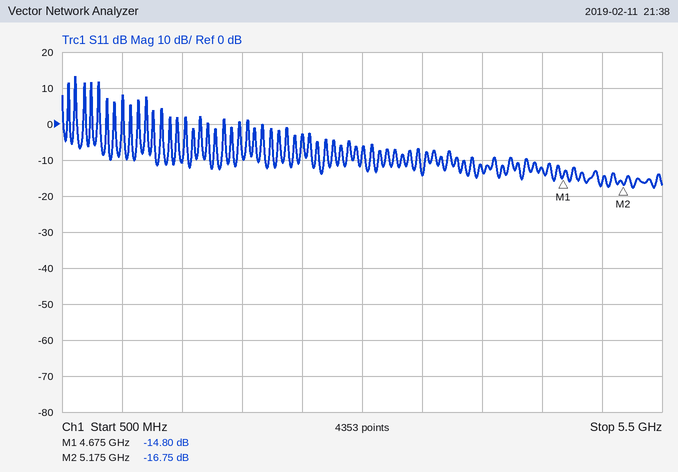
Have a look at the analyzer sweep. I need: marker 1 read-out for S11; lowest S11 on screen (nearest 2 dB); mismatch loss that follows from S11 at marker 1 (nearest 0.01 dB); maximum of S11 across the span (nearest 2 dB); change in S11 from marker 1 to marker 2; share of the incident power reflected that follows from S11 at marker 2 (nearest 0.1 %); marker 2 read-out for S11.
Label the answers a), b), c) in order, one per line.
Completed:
a) -14.80 dB
b) -18 dB
c) 0.15 dB
d) 14 dB
e) -1.95 dB
f) 2.1 %
g) -16.75 dB
